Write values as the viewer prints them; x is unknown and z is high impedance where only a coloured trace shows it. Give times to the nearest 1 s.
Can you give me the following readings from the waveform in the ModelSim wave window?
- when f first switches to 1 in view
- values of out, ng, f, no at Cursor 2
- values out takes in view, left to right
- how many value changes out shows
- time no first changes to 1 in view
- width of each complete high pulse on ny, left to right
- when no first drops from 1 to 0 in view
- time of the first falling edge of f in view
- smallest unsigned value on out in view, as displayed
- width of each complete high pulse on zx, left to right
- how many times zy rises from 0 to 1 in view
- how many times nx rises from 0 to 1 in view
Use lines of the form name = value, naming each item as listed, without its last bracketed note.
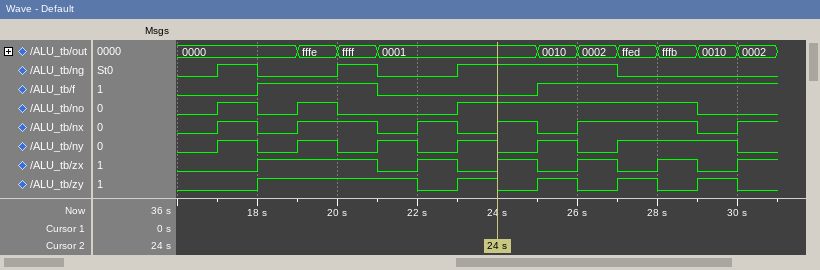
when f first switches to 1 in view = 18 s
values of out, ng, f, no at Cursor 2 = out=0001, ng=1, f=0, no=1
values out takes in view, left to right = 0000, fffe, ffff, 0001, 0010, 0002, ffed, fffb, 0010, 0002
how many value changes out shows = 9
time no first changes to 1 in view = 17 s
width of each complete high pulse on ny, left to right = 1 s, 1 s, 1 s, 1 s, 1 s, 3 s
when no first drops from 1 to 0 in view = 18 s
time of the first falling edge of f in view = 21 s
smallest unsigned value on out in view, as displayed = 0000
width of each complete high pulse on zx, left to right = 3 s, 1 s, 1 s, 1 s, 1 s
how many times zy rises from 0 to 1 in view = 5
how many times nx rises from 0 to 1 in view = 6
